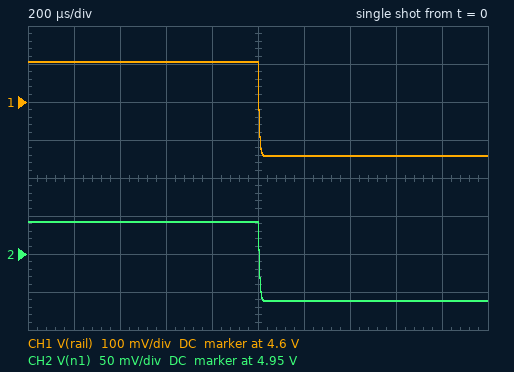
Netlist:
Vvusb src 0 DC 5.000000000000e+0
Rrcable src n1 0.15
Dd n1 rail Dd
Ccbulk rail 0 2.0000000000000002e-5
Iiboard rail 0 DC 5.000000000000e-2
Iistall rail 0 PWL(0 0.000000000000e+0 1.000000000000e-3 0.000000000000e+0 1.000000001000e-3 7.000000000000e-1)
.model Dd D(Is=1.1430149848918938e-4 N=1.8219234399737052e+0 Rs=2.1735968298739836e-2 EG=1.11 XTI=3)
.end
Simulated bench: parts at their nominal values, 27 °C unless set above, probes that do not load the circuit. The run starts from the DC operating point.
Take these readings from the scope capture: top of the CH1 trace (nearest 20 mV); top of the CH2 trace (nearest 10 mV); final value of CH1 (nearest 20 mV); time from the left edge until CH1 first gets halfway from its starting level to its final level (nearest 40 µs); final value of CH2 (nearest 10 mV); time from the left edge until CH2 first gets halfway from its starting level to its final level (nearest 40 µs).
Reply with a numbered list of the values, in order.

1. 4.70 V
2. 4.99 V
3. 4.46 V
4. 1.00 ms
5. 4.89 V
6. 1.00 ms
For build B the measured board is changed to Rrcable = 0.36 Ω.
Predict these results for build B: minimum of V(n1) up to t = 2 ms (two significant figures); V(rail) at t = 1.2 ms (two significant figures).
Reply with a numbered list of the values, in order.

1. 4.7 V
2. 4.3 V
